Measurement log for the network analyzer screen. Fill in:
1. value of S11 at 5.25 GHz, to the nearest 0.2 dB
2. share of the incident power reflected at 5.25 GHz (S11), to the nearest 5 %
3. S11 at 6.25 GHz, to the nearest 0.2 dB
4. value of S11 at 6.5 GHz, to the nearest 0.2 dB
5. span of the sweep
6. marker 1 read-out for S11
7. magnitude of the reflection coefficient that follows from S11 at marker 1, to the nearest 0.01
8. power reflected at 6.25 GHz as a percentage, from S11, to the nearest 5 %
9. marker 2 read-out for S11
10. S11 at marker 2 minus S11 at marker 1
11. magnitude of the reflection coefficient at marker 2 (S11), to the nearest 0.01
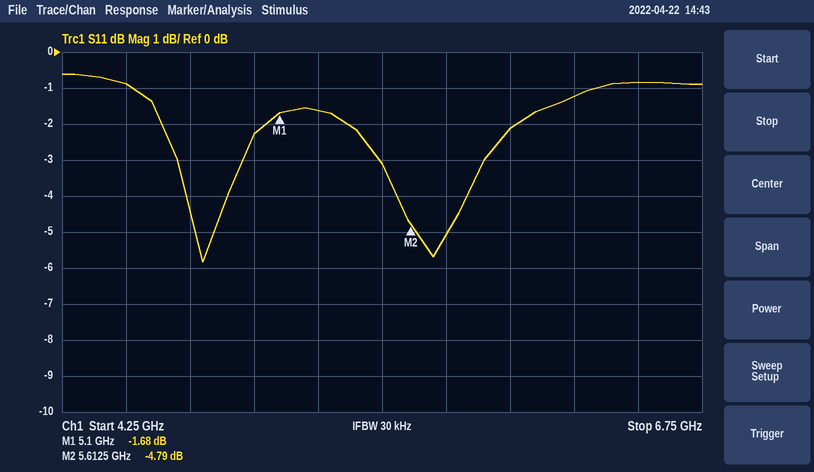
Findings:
-1.6 dB
70 %
-1.2 dB
-0.8 dB
2.5 GHz
-1.68 dB
0.82
75 %
-4.79 dB
-3.11 dB
0.58
